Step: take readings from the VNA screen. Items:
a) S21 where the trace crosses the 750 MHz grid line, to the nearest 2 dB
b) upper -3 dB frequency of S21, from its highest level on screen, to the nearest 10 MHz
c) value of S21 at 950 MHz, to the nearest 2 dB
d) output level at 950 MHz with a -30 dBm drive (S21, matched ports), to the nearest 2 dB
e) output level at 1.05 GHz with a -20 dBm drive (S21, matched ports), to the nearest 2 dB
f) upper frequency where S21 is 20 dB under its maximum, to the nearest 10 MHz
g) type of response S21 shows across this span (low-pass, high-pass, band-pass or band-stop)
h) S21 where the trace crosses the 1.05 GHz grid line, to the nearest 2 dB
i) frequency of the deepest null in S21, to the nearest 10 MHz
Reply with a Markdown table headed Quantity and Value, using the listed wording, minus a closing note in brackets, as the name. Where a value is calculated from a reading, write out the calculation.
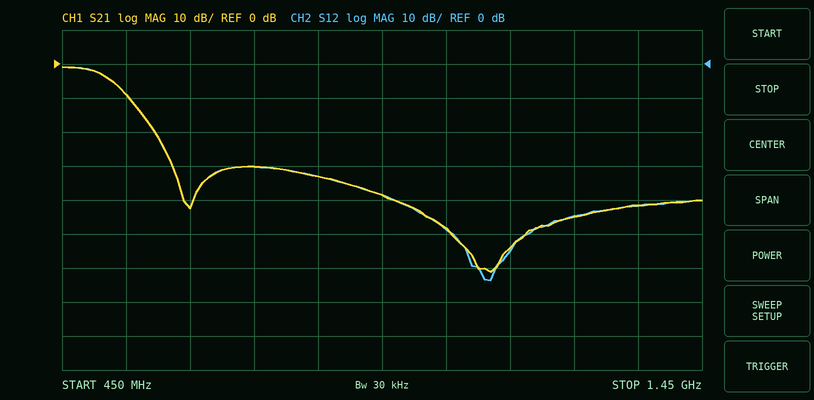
| Quantity | Value |
|---|---|
| S21 where the trace crosses the 750 MHz grid line, to the nearest 2 dB | -30 dB |
| upper -3 dB frequency of S21, from its highest level on screen, to the nearest 10 MHz | 520 MHz |
| value of S21 at 950 MHz, to the nearest 2 dB | -38 dB |
| output level at 950 MHz with a -30 dBm drive (S21, matched ports), to the nearest 2 dB | -30 dBm + (-38 dB) = -68 dBm |
| output level at 1.05 GHz with a -20 dBm drive (S21, matched ports), to the nearest 2 dB | -20 dBm + (-48 dB) = -68 dBm |
| upper frequency where S21 is 20 dB under its maximum, to the nearest 10 MHz | 600 MHz |
| type of response S21 shows across this span | low-pass |
| S21 where the trace crosses the 1.05 GHz grid line, to the nearest 2 dB | -48 dB |
| frequency of the deepest null in S21, to the nearest 10 MHz | 1.12 GHz |
